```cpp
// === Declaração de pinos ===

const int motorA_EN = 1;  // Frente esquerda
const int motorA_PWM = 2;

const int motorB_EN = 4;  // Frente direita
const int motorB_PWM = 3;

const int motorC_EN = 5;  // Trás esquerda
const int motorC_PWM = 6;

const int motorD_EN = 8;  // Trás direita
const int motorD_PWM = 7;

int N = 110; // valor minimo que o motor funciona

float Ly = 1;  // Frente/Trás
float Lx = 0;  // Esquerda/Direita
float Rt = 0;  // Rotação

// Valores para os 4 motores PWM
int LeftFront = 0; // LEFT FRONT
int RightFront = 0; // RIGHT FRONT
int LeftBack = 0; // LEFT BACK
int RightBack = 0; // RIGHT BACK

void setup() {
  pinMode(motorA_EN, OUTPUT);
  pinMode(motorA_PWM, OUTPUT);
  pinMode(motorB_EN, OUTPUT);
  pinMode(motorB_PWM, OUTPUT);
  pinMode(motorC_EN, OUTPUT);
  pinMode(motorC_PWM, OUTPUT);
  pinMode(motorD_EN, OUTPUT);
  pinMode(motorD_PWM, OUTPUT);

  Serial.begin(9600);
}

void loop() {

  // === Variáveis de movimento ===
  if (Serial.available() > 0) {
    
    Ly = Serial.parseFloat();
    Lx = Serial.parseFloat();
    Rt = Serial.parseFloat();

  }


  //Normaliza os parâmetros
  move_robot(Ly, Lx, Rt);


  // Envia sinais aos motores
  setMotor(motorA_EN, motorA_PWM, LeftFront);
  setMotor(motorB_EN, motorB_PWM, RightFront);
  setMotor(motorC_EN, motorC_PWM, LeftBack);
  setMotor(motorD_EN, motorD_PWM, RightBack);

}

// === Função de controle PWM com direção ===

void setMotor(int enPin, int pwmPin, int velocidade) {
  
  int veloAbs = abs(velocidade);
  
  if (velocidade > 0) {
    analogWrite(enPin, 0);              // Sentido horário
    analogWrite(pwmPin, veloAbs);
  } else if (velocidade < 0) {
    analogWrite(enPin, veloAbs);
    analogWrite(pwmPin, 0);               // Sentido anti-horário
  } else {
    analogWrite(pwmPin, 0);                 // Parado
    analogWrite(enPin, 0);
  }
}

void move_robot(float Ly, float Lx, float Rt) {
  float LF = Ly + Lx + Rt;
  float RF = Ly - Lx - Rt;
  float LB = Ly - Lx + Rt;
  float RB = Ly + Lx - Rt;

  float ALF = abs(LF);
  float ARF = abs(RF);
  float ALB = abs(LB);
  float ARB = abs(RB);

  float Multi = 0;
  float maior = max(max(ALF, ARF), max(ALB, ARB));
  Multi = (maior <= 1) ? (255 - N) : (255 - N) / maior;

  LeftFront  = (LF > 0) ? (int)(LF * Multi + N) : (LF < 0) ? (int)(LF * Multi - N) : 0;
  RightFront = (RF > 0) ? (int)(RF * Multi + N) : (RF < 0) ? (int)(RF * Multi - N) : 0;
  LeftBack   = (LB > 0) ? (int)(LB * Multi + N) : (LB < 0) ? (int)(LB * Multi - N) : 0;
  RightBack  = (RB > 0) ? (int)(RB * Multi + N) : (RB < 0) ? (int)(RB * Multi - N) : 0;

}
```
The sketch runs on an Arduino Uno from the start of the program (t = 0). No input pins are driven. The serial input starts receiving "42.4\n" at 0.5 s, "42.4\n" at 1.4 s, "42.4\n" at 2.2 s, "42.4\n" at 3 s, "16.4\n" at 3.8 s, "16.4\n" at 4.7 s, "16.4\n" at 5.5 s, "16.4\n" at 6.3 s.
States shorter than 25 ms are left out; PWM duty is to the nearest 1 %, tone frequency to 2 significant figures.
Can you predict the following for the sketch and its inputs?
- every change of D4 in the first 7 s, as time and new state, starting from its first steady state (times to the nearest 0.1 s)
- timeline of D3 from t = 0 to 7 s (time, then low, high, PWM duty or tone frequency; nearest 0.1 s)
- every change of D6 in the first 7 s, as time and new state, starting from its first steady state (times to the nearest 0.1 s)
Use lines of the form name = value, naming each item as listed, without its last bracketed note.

every change of D4 in the first 7 s, as time and new state, starting from its first steady state = 0 s low; 2.2 s high; 4.7 s low
timeline of D3 from t = 0 to 7 s = 0 s high; 2.2 s low; 4.7 s PWM 50 %
every change of D6 in the first 7 s, as time and new state, starting from its first steady state = 0 s high; 2.2 s PWM 62 %; 4.7 s PWM 75 %
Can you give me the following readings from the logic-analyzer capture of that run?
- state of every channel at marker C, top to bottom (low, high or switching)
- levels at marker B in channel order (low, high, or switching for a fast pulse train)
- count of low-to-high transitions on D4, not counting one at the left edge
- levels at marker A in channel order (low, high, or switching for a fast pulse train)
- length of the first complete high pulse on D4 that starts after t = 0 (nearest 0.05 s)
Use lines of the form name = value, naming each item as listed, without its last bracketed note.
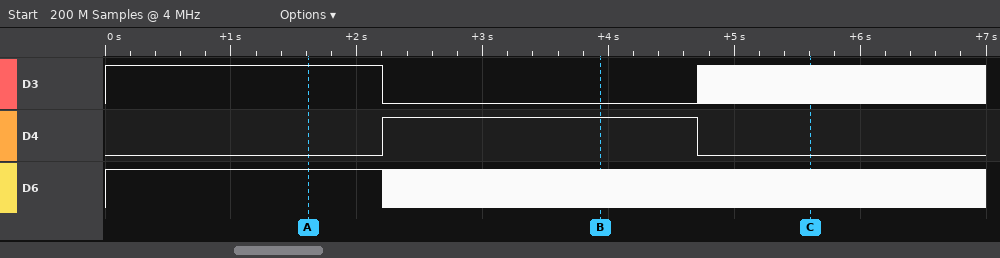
state of every channel at marker C, top to bottom = D3 switching, D4 low, D6 switching
levels at marker B in channel order = D3 low, D4 high, D6 switching
count of low-to-high transitions on D4, not counting one at the left edge = 1
levels at marker A in channel order = D3 high, D4 low, D6 high
length of the first complete high pulse on D4 that starts after t = 0 = 2.50 s
